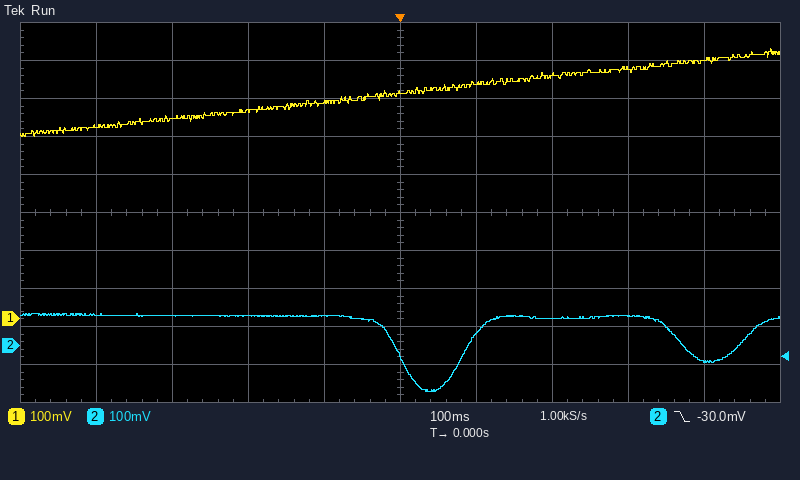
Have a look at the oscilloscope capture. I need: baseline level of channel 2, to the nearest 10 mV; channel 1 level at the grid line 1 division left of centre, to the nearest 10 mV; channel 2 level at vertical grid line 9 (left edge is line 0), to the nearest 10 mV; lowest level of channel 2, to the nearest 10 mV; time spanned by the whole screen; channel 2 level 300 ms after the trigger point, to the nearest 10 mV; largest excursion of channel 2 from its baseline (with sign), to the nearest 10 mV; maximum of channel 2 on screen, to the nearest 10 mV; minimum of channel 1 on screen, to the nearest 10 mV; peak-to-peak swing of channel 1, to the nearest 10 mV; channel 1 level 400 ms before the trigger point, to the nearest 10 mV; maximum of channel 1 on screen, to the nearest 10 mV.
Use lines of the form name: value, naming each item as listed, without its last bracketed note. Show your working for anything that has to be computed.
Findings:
baseline level of channel 2, to the nearest 10 mV: 80 mV
channel 1 level at the grid line 1 division left of centre, to the nearest 10 mV: 570 mV
channel 2 level at vertical grid line 9 (left edge is line 0), to the nearest 10 mV: -40 mV
lowest level of channel 2, to the nearest 10 mV: -120 mV
time spanned by the whole screen: 1 s
channel 2 level 300 ms after the trigger point, to the nearest 10 mV: 80 mV
largest excursion of channel 2 from its baseline (with sign), to the nearest 10 mV: -120 mV − (80 mV) = -200 mV
maximum of channel 2 on screen, to the nearest 10 mV: 80 mV
minimum of channel 1 on screen, to the nearest 10 mV: 480 mV
peak-to-peak swing of channel 1, to the nearest 10 mV: 710 mV − (480 mV) = 230 mV
channel 1 level 400 ms before the trigger point, to the nearest 10 mV: 510 mV
maximum of channel 1 on screen, to the nearest 10 mV: 710 mV
